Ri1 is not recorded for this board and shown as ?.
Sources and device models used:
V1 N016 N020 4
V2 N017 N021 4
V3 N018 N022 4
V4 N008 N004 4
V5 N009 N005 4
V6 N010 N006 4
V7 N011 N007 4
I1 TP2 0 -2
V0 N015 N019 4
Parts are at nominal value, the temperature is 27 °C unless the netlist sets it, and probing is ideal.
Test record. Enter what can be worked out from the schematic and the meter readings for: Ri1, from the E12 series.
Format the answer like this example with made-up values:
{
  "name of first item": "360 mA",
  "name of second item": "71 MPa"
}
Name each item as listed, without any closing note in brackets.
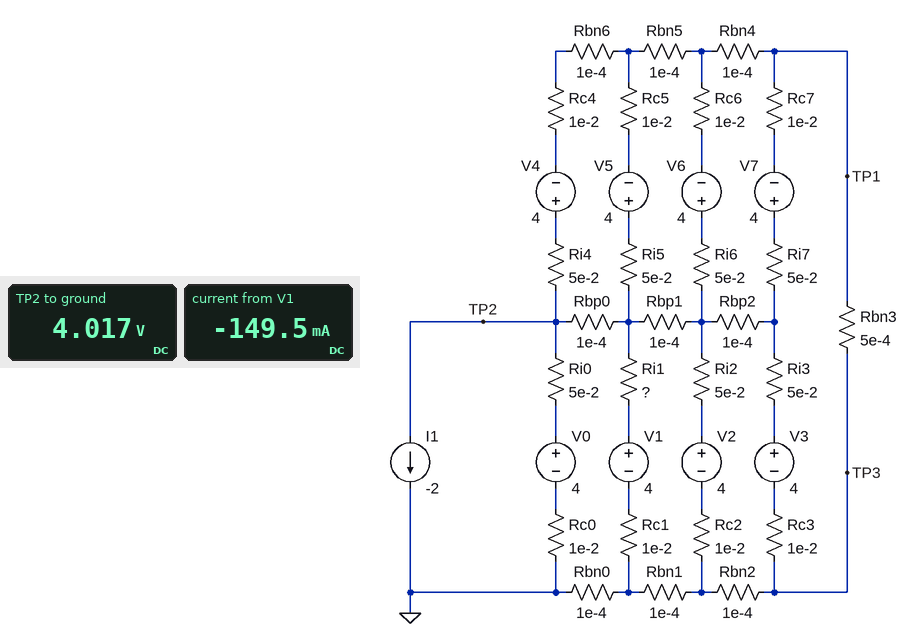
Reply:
{
  "Ri1, from the E12 series": "0.1 Ω"
}
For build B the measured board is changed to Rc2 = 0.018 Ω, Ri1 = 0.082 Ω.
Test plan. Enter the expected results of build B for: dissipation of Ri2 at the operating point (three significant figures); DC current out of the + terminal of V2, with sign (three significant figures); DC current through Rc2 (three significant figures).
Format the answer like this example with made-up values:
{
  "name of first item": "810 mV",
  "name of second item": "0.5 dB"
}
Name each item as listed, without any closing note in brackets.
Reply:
{
  "dissipation of Ri2 at the operating point": "2.84 mW",
  "DC current out of the + terminal of V2, with sign": "-238 mA",
  "DC current through Rc2": "238 mA"
}
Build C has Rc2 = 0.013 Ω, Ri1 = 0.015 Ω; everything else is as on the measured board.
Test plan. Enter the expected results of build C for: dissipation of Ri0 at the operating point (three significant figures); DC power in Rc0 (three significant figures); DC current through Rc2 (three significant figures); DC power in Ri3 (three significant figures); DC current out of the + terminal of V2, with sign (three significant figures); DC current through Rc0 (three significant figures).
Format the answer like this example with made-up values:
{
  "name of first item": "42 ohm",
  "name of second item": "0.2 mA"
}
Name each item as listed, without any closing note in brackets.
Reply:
{
  "dissipation of Ri0 at the operating point": "2.53 mW",
  "DC power in Rc0": "506 µW",
  "DC current through Rc2": "206 mA",
  "DC power in Ri3": "2.28 mW",
  "DC current out of the + terminal of V2, with sign": "-206 mA",
  "DC current through Rc0": "225 mA"
}
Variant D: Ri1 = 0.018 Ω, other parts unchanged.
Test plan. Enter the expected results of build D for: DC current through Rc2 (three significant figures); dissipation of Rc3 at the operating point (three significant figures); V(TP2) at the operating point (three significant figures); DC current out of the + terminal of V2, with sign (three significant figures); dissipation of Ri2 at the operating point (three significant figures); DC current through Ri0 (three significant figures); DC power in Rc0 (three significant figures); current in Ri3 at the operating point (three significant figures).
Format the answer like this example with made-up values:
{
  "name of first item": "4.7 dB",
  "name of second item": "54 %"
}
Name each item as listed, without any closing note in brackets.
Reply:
{
  "DC current through Rc2": "221 mA",
  "dissipation of Rc3 at the operating point": "478 µW",
  "V(TP2) at the operating point": "4.01 V",
  "DC current out of the + terminal of V2, with sign": "-221 mA",
  "dissipation of Ri2 at the operating point": "2.44 mW",
  "DC current through Ri0": "230 mA",
  "DC power in Rc0": "530 µW",
  "current in Ri3 at the operating point": "219 mA"
}
